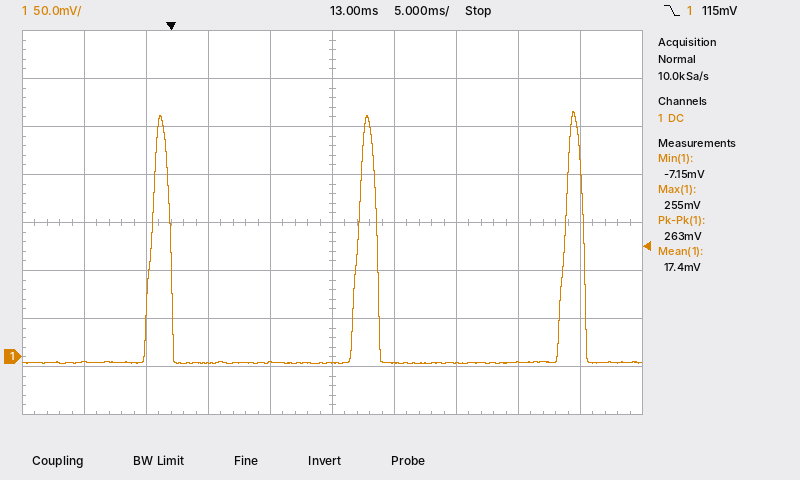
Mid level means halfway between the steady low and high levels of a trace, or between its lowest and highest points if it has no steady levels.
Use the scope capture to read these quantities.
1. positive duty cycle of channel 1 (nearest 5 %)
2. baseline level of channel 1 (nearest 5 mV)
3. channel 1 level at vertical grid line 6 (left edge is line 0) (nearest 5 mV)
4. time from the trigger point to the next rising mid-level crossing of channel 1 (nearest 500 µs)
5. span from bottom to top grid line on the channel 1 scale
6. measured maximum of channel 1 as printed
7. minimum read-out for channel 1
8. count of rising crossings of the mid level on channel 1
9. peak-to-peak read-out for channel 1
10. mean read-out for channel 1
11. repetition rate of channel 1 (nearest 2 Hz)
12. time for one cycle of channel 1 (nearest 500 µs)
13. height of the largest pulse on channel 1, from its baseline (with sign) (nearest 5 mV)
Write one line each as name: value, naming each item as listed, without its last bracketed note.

positive duty cycle of channel 1: 10 %
baseline level of channel 1: -5 mV
channel 1 level at vertical grid line 6 (left edge is line 0): -5 mV
time from the trigger point to the next rising mid-level crossing of channel 1: 15.0 ms
span from bottom to top grid line on the channel 1 scale: 400 mV
measured maximum of channel 1 as printed: 255 mV
minimum read-out for channel 1: -7.15 mV
count of rising crossings of the mid level on channel 1: 3
peak-to-peak read-out for channel 1: 263 mV
mean read-out for channel 1: 17.4 mV
repetition rate of channel 1: 60 Hz
time for one cycle of channel 1: 16.5 ms
height of the largest pulse on channel 1, from its baseline (with sign): +260 mV
